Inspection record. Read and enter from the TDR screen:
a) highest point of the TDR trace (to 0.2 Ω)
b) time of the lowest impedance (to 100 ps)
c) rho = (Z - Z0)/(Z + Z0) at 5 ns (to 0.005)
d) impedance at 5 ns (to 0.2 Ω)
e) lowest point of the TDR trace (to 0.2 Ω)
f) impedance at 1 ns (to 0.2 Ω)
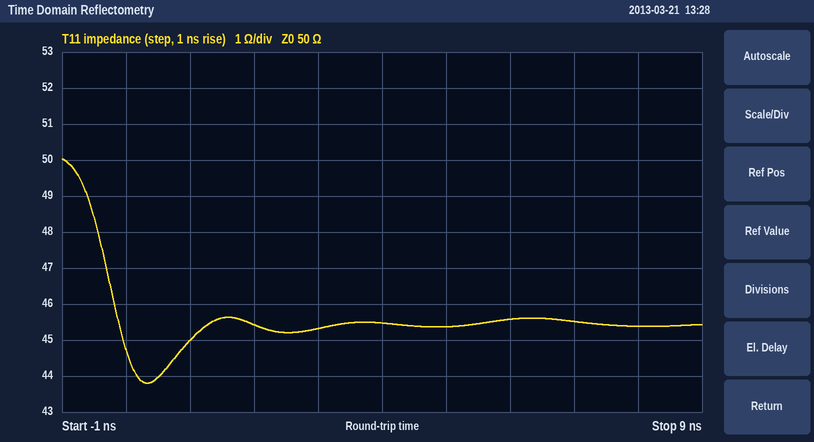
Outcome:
50.0 Ω
300 ps
-0.050
45.4 Ω
43.8 Ω
45.0 Ω
